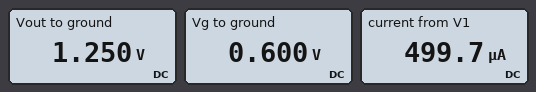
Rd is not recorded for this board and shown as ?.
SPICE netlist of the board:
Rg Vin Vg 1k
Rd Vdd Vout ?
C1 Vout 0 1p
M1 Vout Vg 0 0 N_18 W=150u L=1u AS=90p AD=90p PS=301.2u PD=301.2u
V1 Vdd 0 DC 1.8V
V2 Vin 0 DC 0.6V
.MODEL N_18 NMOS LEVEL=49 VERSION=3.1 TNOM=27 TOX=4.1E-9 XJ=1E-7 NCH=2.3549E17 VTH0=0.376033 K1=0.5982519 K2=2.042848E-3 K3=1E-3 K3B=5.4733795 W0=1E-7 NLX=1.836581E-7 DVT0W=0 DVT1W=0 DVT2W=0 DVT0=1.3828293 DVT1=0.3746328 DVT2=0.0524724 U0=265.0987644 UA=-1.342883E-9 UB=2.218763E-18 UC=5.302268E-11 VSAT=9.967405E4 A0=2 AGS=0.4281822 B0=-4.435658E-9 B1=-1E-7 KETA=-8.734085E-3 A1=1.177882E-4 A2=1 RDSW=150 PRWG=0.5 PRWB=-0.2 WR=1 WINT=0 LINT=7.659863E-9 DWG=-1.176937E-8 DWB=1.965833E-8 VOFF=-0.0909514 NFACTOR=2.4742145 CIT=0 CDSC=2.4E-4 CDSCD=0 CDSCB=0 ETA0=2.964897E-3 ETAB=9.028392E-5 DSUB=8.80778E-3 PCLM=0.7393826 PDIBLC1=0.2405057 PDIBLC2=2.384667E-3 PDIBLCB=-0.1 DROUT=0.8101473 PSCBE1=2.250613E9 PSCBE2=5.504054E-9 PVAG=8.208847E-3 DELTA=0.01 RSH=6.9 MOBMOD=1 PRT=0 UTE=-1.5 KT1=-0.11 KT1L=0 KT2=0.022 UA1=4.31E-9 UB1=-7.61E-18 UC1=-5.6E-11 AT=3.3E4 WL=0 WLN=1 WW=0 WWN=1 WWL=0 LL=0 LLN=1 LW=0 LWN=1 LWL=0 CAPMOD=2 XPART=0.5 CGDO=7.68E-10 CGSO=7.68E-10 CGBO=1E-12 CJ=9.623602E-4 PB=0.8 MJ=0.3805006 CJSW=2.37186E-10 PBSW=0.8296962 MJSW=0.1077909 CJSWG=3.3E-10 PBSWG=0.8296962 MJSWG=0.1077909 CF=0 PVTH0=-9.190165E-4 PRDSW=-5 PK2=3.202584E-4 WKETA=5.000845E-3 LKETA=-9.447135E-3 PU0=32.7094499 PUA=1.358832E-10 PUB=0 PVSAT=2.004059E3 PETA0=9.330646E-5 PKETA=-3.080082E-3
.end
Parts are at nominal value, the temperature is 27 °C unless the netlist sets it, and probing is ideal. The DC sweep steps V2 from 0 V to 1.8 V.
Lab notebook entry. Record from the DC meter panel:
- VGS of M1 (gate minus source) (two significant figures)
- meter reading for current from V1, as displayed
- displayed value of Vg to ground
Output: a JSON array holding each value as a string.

["600 mV", "499.7 µA", "0.600 V"]
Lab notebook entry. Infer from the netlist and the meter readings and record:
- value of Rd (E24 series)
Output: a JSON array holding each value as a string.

["1.1 kΩ"]
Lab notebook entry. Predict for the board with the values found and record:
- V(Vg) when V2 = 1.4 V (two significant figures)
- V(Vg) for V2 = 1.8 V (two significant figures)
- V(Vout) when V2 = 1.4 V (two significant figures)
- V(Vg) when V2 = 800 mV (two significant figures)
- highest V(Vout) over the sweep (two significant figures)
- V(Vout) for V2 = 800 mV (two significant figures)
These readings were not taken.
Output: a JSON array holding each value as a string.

["1.4 V", "1.8 V", "67 mV", "800 mV", "1.8 V", "160 mV"]
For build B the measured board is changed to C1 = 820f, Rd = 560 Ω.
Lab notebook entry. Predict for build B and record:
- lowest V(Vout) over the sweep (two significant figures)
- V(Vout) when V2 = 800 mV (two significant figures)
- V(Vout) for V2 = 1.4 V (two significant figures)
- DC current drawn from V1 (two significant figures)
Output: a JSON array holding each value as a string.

["110 mV", "660 mV", "130 mV", "510 µA"]
